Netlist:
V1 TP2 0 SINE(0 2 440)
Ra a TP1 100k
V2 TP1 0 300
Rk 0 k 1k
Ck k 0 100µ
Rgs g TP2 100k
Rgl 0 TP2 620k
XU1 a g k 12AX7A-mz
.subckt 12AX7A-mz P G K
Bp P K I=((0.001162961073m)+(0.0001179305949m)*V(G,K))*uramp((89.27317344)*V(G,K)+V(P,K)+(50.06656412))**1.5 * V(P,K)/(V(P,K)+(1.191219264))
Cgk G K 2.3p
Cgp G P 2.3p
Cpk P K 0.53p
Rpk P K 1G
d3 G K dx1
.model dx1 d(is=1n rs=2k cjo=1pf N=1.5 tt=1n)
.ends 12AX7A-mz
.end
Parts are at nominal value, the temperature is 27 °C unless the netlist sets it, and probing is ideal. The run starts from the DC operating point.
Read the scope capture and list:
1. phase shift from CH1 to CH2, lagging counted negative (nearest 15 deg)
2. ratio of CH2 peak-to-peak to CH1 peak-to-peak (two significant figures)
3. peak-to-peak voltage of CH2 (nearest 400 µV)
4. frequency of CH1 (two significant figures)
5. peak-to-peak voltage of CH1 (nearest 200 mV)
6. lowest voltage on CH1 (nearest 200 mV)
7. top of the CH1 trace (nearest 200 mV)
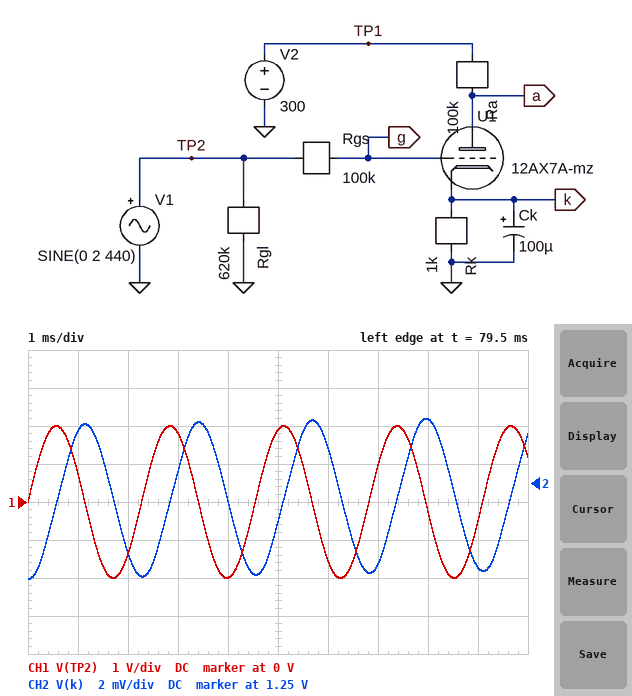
-90 deg
0.0021
8.4 mV
440 Hz
4.0 V
-2.0 V
2.0 V
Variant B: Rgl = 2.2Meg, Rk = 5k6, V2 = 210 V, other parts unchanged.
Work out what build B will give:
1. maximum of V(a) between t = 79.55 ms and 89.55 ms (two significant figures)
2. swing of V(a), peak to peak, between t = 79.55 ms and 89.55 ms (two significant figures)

210 V
140 V
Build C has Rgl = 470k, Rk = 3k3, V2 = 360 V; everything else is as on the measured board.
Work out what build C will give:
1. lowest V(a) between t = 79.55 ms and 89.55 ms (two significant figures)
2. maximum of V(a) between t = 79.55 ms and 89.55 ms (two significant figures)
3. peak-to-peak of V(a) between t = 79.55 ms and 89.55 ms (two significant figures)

160 V
360 V
200 V
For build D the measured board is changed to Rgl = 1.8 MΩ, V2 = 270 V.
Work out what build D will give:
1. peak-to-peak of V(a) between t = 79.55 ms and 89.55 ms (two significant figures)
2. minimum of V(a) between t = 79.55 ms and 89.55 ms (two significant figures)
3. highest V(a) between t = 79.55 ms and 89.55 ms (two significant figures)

190 V
65 V
260 V
